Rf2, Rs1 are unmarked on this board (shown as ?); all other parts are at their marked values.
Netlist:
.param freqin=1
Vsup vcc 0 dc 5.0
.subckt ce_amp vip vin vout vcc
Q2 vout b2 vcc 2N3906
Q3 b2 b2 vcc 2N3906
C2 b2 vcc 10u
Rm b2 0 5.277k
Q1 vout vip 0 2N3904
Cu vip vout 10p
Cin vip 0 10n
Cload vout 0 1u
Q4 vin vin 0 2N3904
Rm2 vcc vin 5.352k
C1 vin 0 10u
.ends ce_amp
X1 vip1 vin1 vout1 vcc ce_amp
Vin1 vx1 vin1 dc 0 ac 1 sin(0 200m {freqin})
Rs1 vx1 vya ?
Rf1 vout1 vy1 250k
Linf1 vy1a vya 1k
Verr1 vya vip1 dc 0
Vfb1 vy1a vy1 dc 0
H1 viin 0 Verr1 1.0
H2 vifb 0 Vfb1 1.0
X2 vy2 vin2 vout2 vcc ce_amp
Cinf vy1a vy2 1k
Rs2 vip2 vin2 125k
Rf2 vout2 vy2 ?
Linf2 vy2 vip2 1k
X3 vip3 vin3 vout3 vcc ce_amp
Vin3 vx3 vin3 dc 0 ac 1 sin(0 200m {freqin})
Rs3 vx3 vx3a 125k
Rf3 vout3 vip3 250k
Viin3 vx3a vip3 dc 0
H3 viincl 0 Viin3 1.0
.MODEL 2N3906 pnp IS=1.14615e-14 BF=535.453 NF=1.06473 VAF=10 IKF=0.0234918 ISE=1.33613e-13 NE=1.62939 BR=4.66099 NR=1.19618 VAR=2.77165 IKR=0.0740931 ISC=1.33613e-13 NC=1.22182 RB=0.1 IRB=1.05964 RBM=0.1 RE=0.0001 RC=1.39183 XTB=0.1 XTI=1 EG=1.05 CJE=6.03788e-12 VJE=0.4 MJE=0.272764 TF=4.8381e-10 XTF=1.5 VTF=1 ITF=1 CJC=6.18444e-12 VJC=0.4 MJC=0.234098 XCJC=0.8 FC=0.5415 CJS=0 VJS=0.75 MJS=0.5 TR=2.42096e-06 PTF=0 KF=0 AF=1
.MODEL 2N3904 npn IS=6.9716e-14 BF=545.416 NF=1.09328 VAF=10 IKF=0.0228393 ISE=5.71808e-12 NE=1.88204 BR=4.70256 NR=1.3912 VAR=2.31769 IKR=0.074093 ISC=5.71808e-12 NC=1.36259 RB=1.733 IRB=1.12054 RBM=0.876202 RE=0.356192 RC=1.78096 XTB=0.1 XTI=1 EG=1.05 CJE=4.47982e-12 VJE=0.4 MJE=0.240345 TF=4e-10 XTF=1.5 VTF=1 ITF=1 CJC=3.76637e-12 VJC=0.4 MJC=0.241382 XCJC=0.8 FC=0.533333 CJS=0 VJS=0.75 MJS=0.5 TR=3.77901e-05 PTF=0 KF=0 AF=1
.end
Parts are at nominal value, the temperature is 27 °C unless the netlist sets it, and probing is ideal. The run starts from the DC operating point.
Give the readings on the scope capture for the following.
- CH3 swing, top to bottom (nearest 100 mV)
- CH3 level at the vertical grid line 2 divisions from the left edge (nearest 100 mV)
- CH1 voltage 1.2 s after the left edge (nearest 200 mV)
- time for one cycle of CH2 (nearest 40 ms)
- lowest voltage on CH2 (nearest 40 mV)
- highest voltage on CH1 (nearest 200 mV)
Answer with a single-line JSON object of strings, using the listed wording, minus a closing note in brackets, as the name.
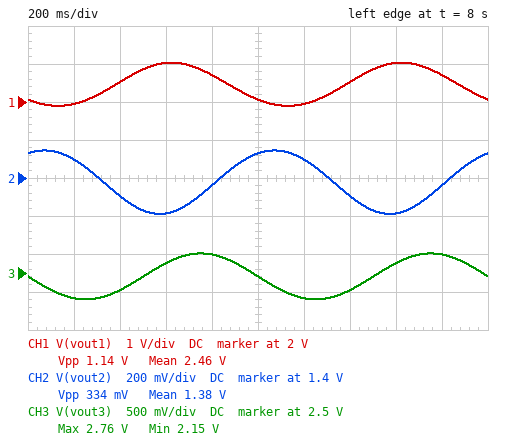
{"CH3 swing, top to bottom": "600 mV", "CH3 level at the vertical grid line 2 divisions from the left edge": "2.3 V", "CH1 voltage 1.2 s after the left edge": "2.0 V", "time for one cycle of CH2": "1.00 s", "lowest voltage on CH2": "1.20 V", "highest voltage on CH1": "3.0 V"}
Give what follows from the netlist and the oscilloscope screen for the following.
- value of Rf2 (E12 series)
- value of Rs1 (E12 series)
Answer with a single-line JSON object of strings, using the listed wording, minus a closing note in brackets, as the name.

{"value of Rf2": "82 kΩ", "value of Rs1": "180 kΩ"}
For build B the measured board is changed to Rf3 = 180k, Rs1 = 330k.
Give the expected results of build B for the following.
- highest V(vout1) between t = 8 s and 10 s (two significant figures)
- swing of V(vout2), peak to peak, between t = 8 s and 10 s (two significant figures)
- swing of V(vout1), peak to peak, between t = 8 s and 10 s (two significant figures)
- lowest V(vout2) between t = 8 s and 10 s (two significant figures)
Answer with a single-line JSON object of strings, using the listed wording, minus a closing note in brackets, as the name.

{"highest V(vout1) between t = 8 s and 10 s": "2.8 V", "swing of V(vout2), peak to peak, between t = 8 s and 10 s": "180 mV", "swing of V(vout1), peak to peak, between t = 8 s and 10 s": "620 mV", "lowest V(vout2) between t = 8 s and 10 s": "1.3 V"}
